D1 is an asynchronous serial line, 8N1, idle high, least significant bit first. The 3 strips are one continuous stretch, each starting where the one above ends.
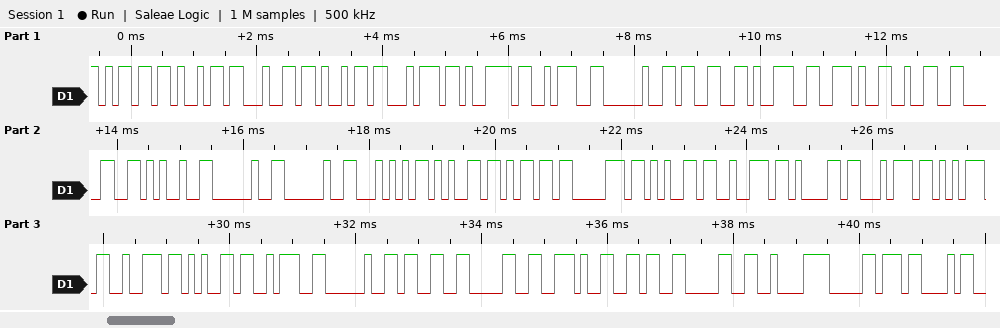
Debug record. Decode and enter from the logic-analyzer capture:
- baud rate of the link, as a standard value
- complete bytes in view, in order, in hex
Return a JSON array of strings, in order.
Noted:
["9600 baud", "0x6D 0x69 0x64 0x69 0x74 0x79 0x3A 0x20 0x33 0x39 0x2E 0x32 0x30 0x25 0x20 0x20 0x54 0x65 0x6D 0x70 0x65 0x72 0x61 0x74 0x75 0x72 0x65 0x3A 0x20 0x33 0x30 0x2E 0x36 0x30 0xC2 0xB0 0x43"]
